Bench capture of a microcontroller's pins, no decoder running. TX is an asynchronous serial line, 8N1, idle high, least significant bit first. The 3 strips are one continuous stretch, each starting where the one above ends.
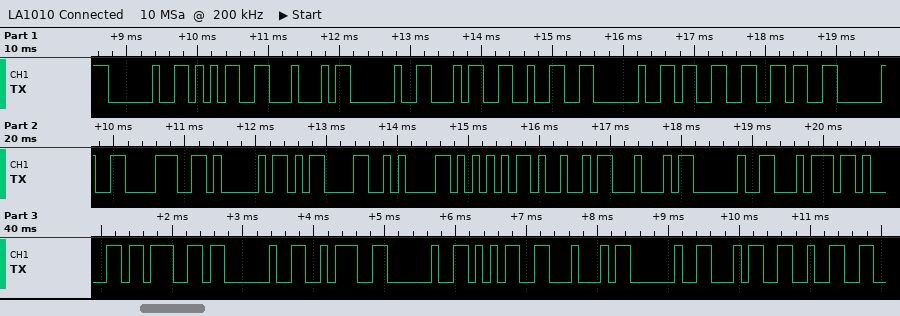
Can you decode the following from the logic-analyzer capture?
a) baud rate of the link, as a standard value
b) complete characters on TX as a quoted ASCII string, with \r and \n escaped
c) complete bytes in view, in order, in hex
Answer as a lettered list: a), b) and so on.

a) 9600 baud
b) " 5D 42 36 8A\r\nUID tag : 5D 42"
c) 20 35 44 20 34 32 20 33 36 20 38 41 0D 0A 55 49 44 20 74 61 67 20 3A 20 35 44 20 34 32
